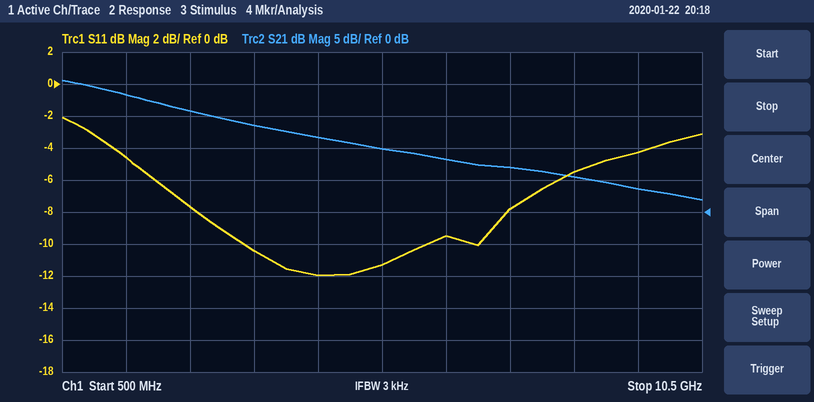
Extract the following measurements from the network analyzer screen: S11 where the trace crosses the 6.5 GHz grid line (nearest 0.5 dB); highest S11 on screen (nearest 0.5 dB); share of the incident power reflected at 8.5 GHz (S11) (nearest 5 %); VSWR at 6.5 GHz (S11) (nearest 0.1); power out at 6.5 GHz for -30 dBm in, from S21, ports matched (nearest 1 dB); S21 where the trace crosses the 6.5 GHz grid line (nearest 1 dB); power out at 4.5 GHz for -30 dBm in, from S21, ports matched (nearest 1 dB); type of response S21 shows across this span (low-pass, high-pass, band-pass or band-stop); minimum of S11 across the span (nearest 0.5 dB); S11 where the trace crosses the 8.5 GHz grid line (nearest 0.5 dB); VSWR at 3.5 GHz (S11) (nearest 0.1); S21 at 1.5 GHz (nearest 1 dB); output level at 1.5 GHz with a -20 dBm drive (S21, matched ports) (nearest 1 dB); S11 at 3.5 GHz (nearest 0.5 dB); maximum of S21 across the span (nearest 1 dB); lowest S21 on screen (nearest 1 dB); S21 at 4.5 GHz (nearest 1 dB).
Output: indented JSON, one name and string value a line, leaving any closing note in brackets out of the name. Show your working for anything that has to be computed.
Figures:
{
  "S11 where the trace crosses the 6.5 GHz grid line": "-9.5 dB",
  "highest S11 on screen": "-2.0 dB",
  "share of the incident power reflected at 8.5 GHz (S11)": "10^(-5.5/10) ≈ 28.2 %, so 30 % to the nearest 5 %",
  "VSWR at 6.5 GHz (S11)": "|Γ| = 10^(-9.5/20) = 0.3350; VSWR = (1 + 0.3350)/(1 − 0.3350) ≈ 2.0",
  "power out at 6.5 GHz for -30 dBm in, from S21, ports matched": "-30 dBm + (8 dB) = -22 dBm",
  "S21 where the trace crosses the 6.5 GHz grid line": "8 dB",
  "power out at 4.5 GHz for -30 dBm in, from S21, ports matched": "-30 dBm + (12 dB) = -18 dBm",
  "type of response S21 shows across this span": "low-pass",
  "minimum of S11 across the span": "-12.0 dB",
  "S11 where the trace crosses the 8.5 GHz grid line": "-5.5 dB",
  "VSWR at 3.5 GHz (S11)": "|Γ| = 10^(-10.5/20) = 0.2985; VSWR = (1 + 0.2985)/(1 − 0.2985) ≈ 1.9",
  "S21 at 1.5 GHz": "18 dB",
  "output level at 1.5 GHz with a -20 dBm drive (S21, matched ports)": "-20 dBm + (18 dB) = -2 dBm",
  "S11 at 3.5 GHz": "-10.5 dB",
  "maximum of S21 across the span": "21 dB",
  "lowest S21 on screen": "2 dB",
  "S21 at 4.5 GHz": "12 dB"
}
